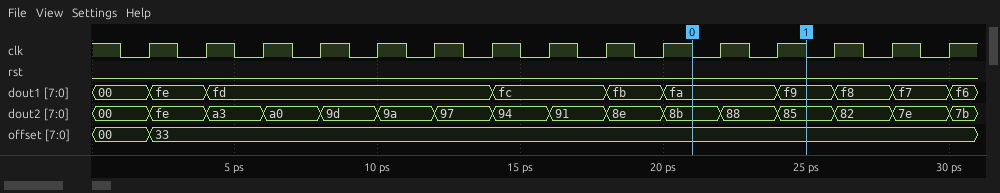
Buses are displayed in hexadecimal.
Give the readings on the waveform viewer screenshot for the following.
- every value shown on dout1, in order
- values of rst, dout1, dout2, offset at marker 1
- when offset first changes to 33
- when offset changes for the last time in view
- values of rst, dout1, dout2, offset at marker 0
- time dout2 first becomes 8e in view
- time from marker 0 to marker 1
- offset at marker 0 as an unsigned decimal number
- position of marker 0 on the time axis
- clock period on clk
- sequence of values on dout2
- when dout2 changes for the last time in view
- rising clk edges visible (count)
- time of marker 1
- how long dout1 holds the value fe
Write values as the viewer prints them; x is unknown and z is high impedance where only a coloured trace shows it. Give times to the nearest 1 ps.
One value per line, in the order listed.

00, fe, fd, fc, fb, fa, f9, f8, f7, f6
rst=0, dout1=f9, dout2=85, offset=33
2 ps
2 ps
rst=0, dout1=fa, dout2=8b, offset=33
18 ps
4 ps
51
21 ps
2 ps
00, fe, a3, a0, 9d, 9a, 97, 94, 91, 8e, 8b, 88, 85, 82, 7e, 7b
30 ps
15
25 ps
2 ps
